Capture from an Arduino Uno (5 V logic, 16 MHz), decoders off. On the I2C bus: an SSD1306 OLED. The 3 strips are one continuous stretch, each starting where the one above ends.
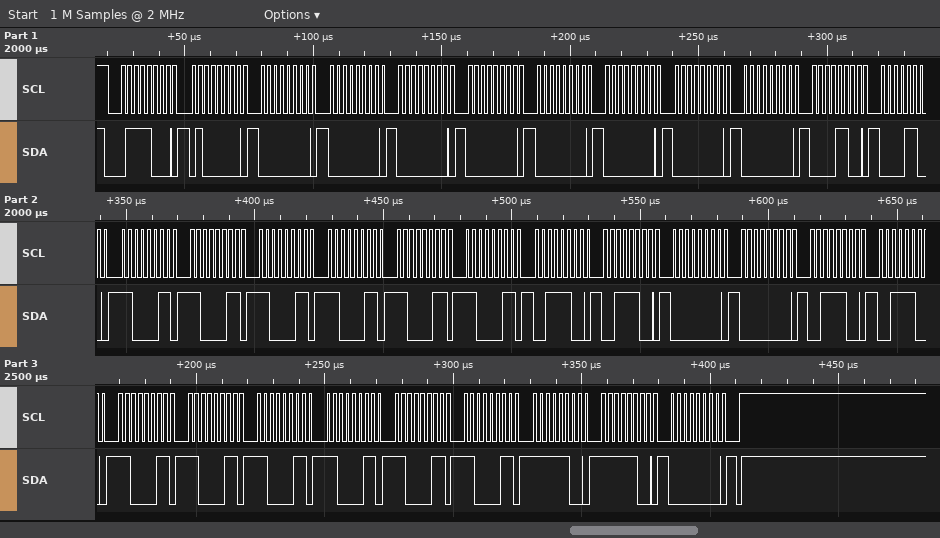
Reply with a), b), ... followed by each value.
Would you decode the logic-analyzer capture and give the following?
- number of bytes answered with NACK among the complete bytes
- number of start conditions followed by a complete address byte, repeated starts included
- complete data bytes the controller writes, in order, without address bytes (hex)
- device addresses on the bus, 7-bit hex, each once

a) 0
b) 1
c) 40 00 00 00 00 00 00 00 00 0C 0C C3 C3 C3 C3 C3 C3 3C 3C 00 00 3C 3C C3 C3 C3 C3 C3 C3 FC FC 00
d) 0x3C
